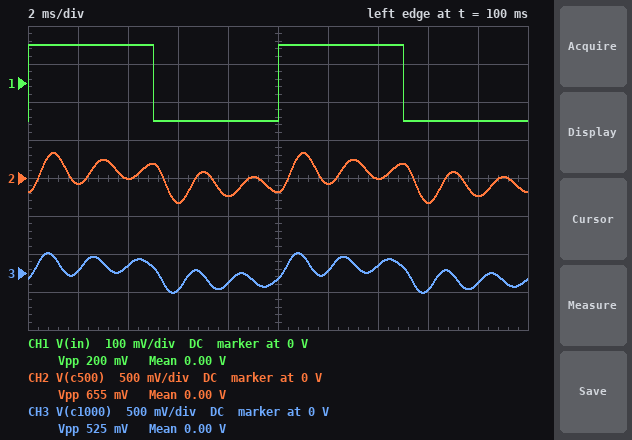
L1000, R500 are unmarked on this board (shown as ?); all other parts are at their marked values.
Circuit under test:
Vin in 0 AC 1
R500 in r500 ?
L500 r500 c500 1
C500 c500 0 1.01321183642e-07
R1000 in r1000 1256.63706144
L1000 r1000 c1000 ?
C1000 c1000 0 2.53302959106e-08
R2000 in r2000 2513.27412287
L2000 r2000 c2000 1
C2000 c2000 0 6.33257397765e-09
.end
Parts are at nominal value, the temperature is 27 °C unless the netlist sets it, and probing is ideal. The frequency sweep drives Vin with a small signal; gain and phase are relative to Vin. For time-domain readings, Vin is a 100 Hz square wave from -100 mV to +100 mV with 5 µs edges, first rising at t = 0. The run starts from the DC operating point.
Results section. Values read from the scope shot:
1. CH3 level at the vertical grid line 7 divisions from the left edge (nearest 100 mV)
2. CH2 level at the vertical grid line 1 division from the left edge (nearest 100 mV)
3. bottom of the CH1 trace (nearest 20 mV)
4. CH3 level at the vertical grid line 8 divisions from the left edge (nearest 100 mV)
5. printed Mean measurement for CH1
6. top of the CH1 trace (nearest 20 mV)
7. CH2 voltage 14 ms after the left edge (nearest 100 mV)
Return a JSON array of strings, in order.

["100 mV", "-100 mV", "-100 mV", "-200 mV", "0.00 V", "100 mV", "0 V"]
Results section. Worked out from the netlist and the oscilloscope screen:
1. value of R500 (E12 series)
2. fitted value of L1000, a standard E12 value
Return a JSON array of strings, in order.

["470 Ω", "3.3 H"]
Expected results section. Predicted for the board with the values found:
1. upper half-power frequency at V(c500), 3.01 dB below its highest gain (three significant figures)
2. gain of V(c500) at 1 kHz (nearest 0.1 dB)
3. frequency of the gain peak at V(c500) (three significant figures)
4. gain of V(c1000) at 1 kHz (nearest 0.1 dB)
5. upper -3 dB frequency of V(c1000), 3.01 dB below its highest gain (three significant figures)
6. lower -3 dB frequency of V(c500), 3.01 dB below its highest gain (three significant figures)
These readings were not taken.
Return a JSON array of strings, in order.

["533 Hz", "-9.6 dB", "497 Hz", "-7.3 dB", "578 Hz", "458 Hz"]
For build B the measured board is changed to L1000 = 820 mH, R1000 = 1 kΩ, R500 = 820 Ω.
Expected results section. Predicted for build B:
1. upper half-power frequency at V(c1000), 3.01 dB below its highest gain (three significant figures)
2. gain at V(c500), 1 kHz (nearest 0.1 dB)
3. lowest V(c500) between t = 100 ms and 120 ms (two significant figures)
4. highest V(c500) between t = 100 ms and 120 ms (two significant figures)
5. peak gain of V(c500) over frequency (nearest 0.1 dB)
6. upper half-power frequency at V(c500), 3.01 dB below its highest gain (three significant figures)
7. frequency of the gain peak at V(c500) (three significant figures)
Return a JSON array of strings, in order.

["1.19 kHz", "-9.7 dB", "-250 mV", "250 mV", "11.7 dB", "553 Hz", "491 Hz"]
